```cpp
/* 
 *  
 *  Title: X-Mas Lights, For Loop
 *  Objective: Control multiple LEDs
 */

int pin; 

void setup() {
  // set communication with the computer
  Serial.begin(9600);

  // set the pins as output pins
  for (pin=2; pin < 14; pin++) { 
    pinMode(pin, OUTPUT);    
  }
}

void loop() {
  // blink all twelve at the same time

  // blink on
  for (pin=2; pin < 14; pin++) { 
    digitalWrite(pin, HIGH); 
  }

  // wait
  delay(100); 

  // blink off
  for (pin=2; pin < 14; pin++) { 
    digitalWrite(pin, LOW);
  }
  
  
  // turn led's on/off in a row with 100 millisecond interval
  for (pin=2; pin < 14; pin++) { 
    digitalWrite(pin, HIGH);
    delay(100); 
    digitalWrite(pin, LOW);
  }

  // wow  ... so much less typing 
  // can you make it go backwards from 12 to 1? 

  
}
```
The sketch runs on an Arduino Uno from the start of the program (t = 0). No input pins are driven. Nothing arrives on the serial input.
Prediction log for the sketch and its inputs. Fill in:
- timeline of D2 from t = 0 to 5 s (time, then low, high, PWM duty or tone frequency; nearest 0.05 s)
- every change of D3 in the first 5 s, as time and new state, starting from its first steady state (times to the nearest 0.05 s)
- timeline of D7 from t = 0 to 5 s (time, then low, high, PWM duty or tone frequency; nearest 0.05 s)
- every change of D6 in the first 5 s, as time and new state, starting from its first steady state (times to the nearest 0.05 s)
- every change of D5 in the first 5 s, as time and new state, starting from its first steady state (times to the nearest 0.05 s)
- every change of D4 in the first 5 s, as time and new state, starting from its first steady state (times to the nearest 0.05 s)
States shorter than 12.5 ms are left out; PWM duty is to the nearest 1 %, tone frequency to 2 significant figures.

0 s high; 0.2 s low; 1.3 s high; 1.5 s low; 2.6 s high; 2.8 s low; 3.9 s high; 4.1 s low
0 s high; 0.1 s low; 0.2 s high; 0.3 s low; 1.3 s high; 1.4 s low; 1.5 s high; 1.6 s low; 2.6 s high; 2.7 s low; 2.8 s high; 2.9 s low; 3.9 s high; 4 s low; 4.1 s high; 4.2 s low
0 s high; 0.1 s low; 0.6 s high; 0.7 s low; 1.3 s high; 1.4 s low; 1.9 s high; 2 s low; 2.6 s high; 2.7 s low; 3.2 s high; 3.3 s low; 3.9 s high; 4 s low; 4.5 s high; 4.6 s low
0 s high; 0.1 s low; 0.5 s high; 0.6 s low; 1.3 s high; 1.4 s low; 1.8 s high; 1.9 s low; 2.6 s high; 2.7 s low; 3.1 s high; 3.2 s low; 3.9 s high; 4 s low; 4.4 s high; 4.5 s low
0 s high; 0.1 s low; 0.4 s high; 0.5 s low; 1.3 s high; 1.4 s low; 1.7 s high; 1.8 s low; 2.6 s high; 2.7 s low; 3 s high; 3.1 s low; 3.9 s high; 4 s low; 4.3 s high; 4.4 s low
0 s high; 0.1 s low; 0.3 s high; 0.4 s low; 1.3 s high; 1.4 s low; 1.6 s high; 1.7 s low; 2.6 s high; 2.7 s low; 2.9 s high; 3 s low; 3.9 s high; 4 s low; 4.2 s high; 4.3 s low
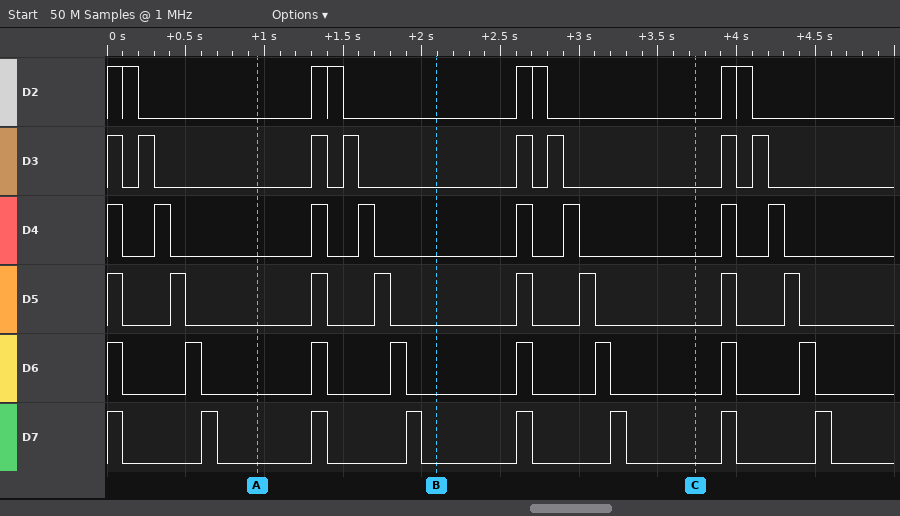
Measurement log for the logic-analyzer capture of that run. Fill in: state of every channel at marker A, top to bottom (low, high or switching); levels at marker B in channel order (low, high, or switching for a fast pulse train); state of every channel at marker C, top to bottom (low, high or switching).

D2 low, D3 low, D4 low, D5 low, D6 low, D7 low
D2 low, D3 low, D4 low, D5 low, D6 low, D7 low
D2 low, D3 low, D4 low, D5 low, D6 low, D7 low
